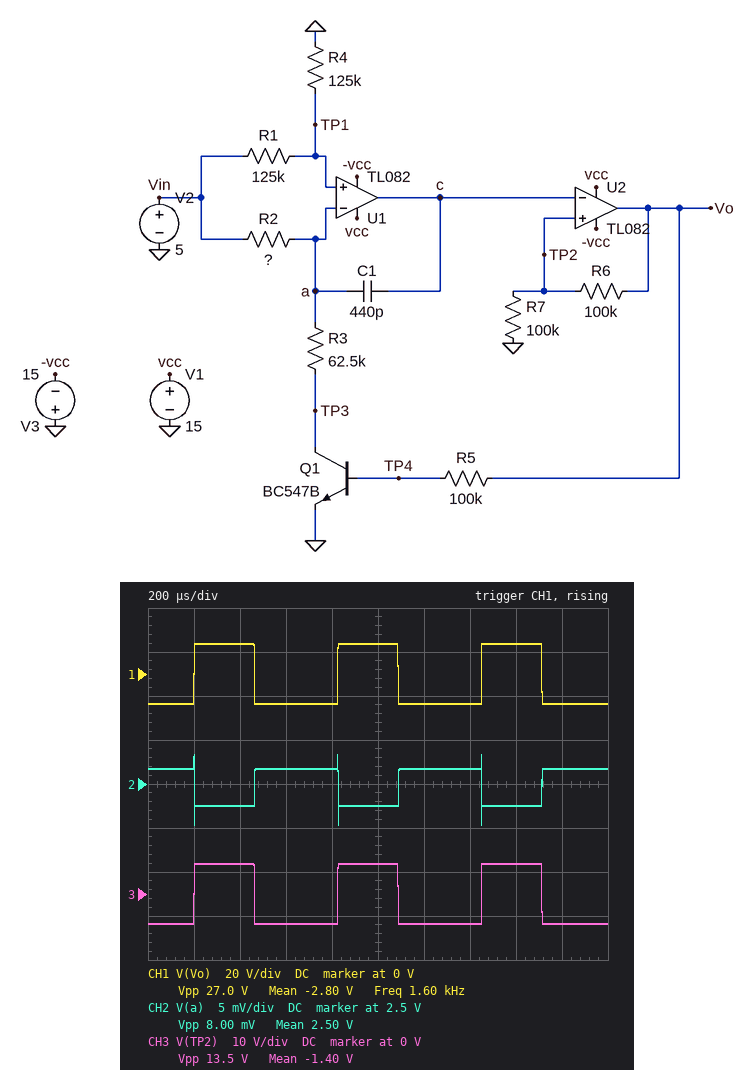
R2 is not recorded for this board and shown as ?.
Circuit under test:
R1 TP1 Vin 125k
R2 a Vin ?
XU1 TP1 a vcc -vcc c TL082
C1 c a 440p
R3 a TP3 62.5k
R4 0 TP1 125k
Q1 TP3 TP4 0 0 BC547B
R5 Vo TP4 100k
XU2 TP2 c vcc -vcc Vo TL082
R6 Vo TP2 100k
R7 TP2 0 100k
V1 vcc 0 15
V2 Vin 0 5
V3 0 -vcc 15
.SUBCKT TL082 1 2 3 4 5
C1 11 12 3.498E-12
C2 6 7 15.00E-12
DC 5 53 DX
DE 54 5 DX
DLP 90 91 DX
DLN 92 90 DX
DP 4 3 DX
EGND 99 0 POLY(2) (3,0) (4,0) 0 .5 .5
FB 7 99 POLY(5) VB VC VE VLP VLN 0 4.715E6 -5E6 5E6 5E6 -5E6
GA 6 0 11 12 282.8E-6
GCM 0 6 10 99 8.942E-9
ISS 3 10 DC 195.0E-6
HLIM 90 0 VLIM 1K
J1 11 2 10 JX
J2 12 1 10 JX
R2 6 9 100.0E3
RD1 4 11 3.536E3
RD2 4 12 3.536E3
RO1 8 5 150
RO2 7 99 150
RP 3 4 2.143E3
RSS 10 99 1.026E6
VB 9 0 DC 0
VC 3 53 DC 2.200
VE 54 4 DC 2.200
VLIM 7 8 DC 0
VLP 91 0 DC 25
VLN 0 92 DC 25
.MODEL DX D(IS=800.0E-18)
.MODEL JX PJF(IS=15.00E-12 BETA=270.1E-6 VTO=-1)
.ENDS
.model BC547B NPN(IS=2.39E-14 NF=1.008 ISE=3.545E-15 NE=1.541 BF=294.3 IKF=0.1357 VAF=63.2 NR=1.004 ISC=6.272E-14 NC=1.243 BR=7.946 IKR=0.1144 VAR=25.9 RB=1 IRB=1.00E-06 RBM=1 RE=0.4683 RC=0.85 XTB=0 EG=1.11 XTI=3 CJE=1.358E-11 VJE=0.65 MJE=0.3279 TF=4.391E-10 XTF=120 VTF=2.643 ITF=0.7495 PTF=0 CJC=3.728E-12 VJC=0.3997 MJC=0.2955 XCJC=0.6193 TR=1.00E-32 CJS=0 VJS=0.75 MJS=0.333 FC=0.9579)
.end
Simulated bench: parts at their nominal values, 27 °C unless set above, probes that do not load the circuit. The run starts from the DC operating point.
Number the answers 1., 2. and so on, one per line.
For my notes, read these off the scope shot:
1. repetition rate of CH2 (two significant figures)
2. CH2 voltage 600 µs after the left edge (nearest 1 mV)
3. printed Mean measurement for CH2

1. 1.6 kHz
2. 2.502 V
3. 2.50 V
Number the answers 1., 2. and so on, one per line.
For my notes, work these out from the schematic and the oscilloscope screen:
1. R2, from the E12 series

1. 150 kΩ
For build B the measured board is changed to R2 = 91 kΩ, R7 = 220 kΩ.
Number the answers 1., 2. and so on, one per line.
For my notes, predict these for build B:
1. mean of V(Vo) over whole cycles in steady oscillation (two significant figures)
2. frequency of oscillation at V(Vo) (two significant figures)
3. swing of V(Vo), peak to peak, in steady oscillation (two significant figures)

1. 5.1 V
2. 1.0 kHz
3. 27 V
